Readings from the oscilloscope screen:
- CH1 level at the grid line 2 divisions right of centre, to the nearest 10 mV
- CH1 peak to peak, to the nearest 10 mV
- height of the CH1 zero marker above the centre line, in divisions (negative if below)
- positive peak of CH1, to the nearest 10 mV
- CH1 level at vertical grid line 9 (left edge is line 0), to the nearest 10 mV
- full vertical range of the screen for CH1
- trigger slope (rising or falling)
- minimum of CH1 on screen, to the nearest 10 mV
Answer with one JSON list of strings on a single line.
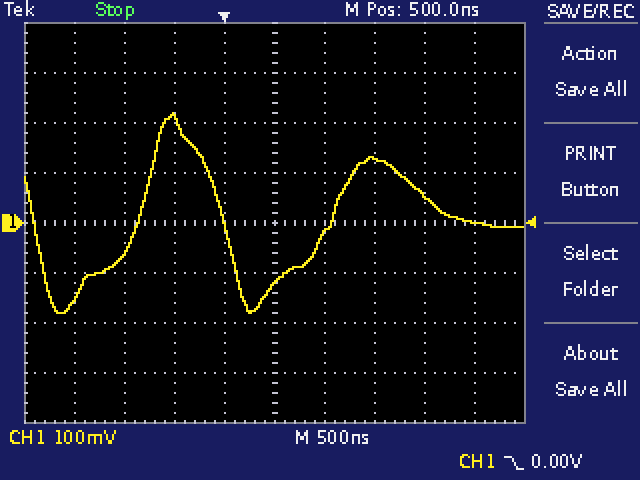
["130 mV", "400 mV", "0.0 div", "220 mV", "0 mV", "800 mV", "falling", "-180 mV"]
